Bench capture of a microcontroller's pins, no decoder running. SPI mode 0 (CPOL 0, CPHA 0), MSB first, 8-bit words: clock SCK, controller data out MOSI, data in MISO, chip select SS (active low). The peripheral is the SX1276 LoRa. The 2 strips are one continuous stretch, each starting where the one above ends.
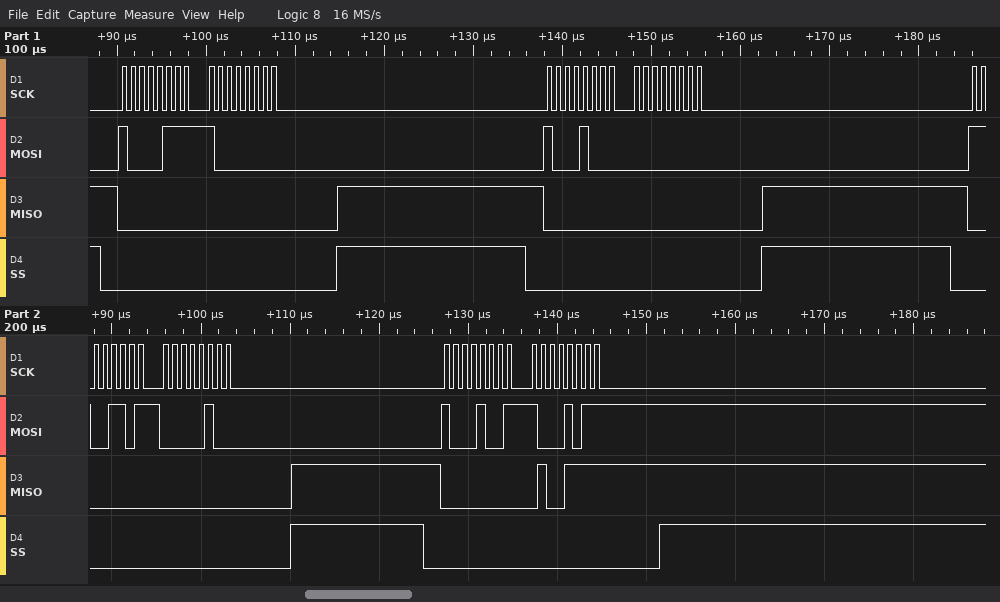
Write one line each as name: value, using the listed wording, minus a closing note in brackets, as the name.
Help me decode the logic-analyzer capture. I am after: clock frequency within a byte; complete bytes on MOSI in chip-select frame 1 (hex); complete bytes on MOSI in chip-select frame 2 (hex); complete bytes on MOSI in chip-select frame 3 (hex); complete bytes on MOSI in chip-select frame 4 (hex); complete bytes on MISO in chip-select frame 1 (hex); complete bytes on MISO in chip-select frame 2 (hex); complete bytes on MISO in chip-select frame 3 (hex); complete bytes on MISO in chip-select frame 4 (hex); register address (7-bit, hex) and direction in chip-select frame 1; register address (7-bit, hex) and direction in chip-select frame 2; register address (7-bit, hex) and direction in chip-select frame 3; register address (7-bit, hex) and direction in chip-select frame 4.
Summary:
clock frequency within a byte: 1 MHz
complete bytes on MOSI in chip-select frame 1: 87 80
complete bytes on MOSI in chip-select frame 2: 88 00
complete bytes on MOSI in chip-select frame 3: CD 04
complete bytes on MOSI in chip-select frame 4: 89 8B
complete bytes on MISO in chip-select frame 1: 00 00
complete bytes on MISO in chip-select frame 2: 00 00
complete bytes on MISO in chip-select frame 3: 00 00
complete bytes on MISO in chip-select frame 4: 00 4F
register address (7-bit, hex) and direction in chip-select frame 1: 0x07 write
register address (7-bit, hex) and direction in chip-select frame 2: 0x08 write
register address (7-bit, hex) and direction in chip-select frame 3: 0x4D write
register address (7-bit, hex) and direction in chip-select frame 4: 0x09 write
